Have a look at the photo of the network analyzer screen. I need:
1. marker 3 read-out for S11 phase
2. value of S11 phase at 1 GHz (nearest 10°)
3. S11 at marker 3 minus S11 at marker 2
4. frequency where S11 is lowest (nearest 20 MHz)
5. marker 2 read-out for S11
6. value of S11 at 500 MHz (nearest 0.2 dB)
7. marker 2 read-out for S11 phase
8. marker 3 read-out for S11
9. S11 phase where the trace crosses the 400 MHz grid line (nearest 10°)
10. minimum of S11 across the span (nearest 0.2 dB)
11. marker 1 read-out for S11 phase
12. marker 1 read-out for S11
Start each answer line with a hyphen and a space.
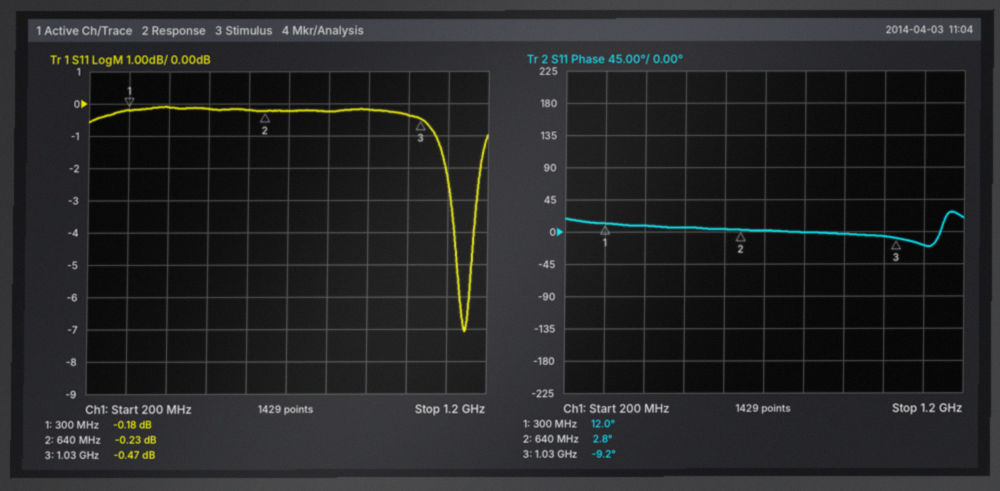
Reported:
- -9.2°
- -10°
- -0.24 dB
- 1.14 GHz
- -0.23 dB
- -0.2 dB
- 2.8°
- -0.47 dB
- 10°
- -7.0 dB
- 12.0°
- -0.18 dB
